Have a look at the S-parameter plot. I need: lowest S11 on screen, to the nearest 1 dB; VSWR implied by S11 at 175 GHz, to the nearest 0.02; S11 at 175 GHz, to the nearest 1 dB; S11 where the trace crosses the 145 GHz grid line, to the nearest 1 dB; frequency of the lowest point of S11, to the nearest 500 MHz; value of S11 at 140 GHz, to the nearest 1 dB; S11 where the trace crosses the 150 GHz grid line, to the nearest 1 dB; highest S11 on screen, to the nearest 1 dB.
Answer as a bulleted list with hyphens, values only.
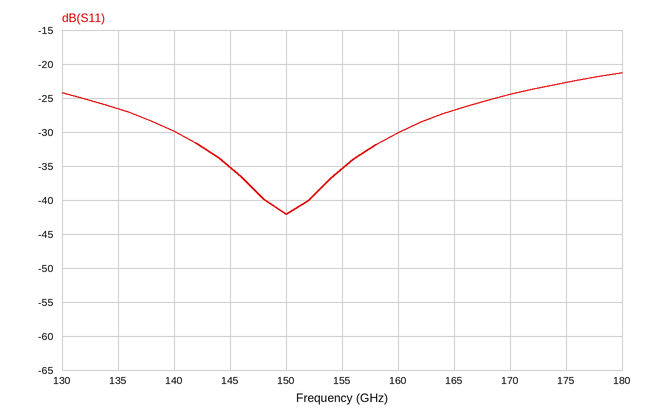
- -42 dB
- 1.16
- -23 dB
- -35 dB
- 150.0 GHz
- -30 dB
- -42 dB
- -21 dB
